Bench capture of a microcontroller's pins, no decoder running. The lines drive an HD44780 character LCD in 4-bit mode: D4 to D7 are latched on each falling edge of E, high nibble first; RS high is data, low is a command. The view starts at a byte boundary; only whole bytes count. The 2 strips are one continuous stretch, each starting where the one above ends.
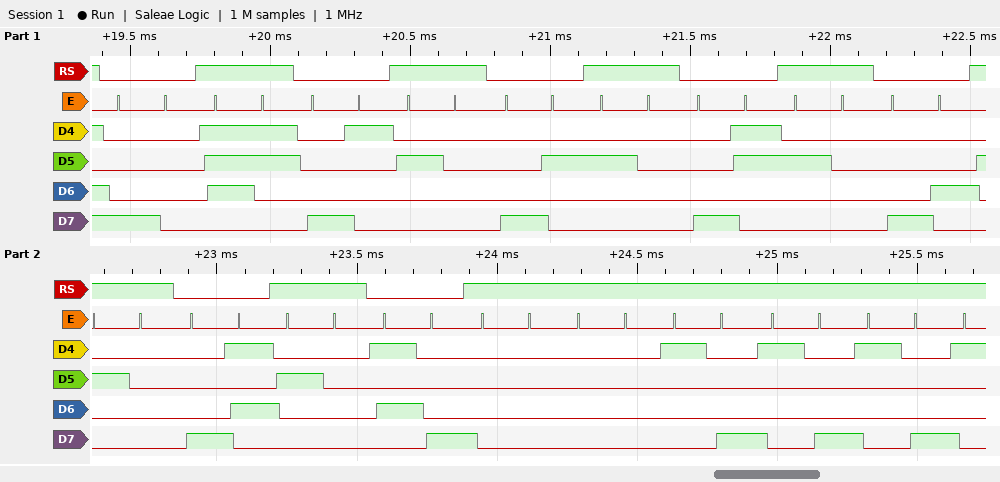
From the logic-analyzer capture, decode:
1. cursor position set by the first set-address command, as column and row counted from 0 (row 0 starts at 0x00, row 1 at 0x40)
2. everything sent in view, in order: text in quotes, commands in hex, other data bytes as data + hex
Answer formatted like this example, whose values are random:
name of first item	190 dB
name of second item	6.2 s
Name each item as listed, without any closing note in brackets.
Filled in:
cursor position set by the first set-address command, as column and row counted from 0	column 0, row 0
everything sent in view, in order: text in quotes, commands in hex, other data bytes as data + hex	0x80 "s" 0x81 " " 0x82 " " 0x83 " " 0x84 " " 0x85 " " 0x58 data 00 00 18 18 18
